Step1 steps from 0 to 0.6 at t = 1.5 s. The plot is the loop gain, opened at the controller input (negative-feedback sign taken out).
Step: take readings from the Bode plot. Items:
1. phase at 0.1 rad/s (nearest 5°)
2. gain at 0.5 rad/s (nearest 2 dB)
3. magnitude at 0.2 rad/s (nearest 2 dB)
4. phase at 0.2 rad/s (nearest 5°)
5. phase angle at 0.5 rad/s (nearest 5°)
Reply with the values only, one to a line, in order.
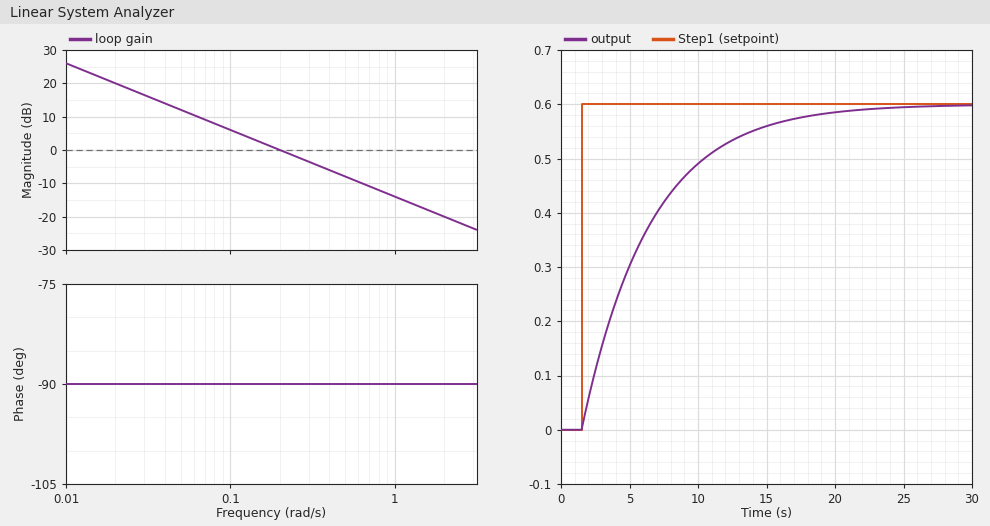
-90°
-8 dB
0 dB
-90°
-90°
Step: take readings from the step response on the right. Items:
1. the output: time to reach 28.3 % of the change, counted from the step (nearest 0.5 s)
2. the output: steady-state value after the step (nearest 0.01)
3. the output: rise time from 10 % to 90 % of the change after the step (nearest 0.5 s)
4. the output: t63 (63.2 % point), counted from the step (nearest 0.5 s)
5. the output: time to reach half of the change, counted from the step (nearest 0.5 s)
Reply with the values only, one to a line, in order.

1.5 s
0.60
11.0 s
5.0 s
3.5 s
